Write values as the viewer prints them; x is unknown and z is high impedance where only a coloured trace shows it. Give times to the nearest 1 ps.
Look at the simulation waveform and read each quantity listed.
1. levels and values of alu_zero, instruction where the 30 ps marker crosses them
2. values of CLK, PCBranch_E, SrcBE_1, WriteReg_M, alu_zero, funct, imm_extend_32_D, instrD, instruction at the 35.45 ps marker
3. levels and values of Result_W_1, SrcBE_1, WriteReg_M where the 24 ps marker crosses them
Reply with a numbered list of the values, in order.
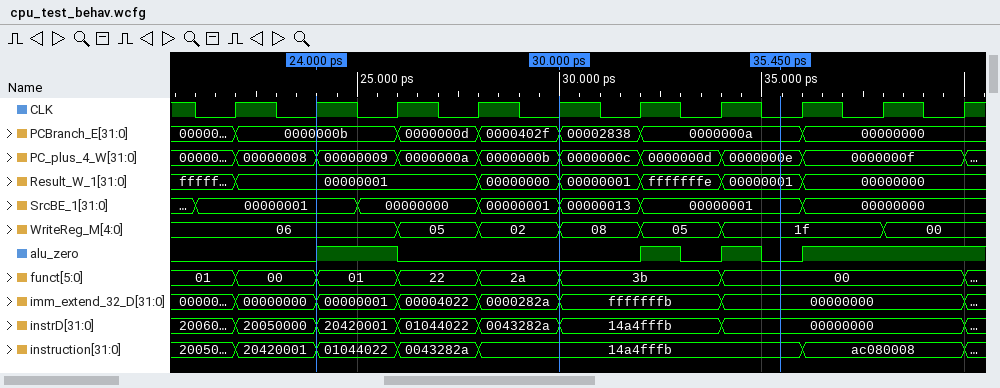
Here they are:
1. alu_zero=0, instruction=14a4fffb
2. CLK=0, PCBranch_E=0000000a, SrcBE_1=00000001, WriteReg_M=1f, alu_zero=0, funct=00, imm_extend_32_D=00000000, instrD=00000000, instruction=14a4fffb
3. Result_W_1=00000001, SrcBE_1=00000001, WriteReg_M=06
